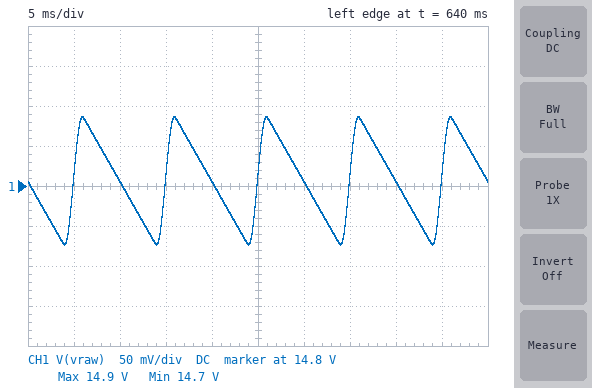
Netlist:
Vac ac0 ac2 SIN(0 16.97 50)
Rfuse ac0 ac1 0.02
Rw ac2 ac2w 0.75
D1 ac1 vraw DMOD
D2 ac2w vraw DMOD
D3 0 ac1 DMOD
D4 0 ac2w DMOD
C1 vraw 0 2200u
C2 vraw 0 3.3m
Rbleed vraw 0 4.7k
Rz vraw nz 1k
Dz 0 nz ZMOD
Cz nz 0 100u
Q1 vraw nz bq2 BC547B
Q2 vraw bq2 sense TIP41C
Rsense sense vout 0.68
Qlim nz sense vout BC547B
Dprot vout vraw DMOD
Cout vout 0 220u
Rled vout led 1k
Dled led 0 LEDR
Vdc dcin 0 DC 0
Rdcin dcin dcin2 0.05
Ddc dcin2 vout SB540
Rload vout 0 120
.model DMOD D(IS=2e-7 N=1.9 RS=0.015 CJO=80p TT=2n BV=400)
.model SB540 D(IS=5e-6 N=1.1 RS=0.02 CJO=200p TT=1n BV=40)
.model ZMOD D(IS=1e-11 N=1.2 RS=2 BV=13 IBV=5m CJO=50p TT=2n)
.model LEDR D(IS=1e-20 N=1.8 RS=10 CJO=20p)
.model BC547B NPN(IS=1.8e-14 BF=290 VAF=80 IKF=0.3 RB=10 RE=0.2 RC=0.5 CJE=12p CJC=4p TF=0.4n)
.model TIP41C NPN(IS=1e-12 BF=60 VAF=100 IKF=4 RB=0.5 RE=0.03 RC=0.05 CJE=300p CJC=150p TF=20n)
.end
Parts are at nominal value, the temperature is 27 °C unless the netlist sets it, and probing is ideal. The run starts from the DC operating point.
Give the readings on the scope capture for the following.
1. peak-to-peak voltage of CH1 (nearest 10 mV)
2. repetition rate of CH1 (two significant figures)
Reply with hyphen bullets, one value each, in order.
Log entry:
- 160 mV
- 100 Hz
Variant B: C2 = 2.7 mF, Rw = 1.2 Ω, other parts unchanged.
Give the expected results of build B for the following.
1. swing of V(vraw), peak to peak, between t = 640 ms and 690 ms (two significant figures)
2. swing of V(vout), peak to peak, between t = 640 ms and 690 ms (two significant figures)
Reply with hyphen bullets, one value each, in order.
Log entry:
- 170 mV
- 1.9 mV
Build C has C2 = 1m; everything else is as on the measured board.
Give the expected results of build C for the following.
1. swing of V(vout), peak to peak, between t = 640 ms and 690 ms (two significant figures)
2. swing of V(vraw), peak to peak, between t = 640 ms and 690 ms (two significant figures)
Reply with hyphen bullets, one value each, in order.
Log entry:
- 2.9 mV
- 270 mV
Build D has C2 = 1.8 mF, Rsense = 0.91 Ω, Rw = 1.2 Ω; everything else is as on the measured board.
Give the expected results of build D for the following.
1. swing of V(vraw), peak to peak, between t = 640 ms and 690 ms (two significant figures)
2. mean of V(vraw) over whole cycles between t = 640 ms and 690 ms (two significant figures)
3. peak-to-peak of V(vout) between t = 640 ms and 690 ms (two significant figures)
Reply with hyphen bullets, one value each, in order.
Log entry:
- 210 mV
- 15 V
- 2.3 mV
